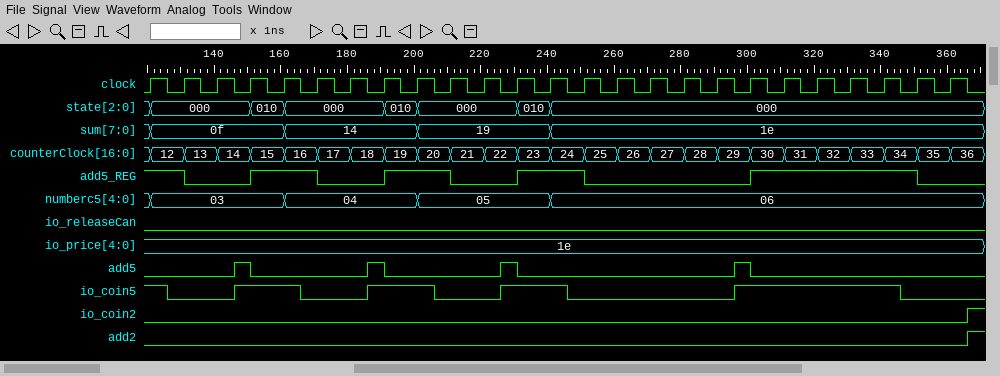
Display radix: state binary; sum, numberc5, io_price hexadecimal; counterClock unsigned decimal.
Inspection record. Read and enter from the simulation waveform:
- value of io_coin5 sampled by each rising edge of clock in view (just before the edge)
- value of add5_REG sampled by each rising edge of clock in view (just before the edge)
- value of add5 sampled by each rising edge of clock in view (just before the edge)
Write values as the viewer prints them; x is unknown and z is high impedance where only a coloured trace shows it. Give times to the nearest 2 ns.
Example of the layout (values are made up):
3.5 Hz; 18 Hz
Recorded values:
1 0 0 1 1 0 0 1 1 0 0 1 1 0 0 0 0 0 1 1 1 1 1 0 0; 1 1 0 0 1 1 0 0 1 1 0 0 1 1 0 0 0 0 0 1 1 1 1 1 0; 0 0 0 1 0 0 0 1 0 0 0 1 0 0 0 0 0 0 1 0 0 0 0 0 0
